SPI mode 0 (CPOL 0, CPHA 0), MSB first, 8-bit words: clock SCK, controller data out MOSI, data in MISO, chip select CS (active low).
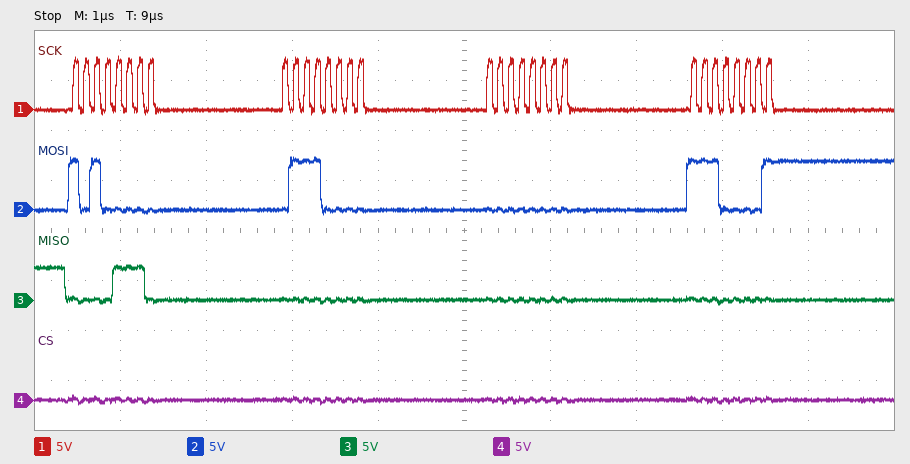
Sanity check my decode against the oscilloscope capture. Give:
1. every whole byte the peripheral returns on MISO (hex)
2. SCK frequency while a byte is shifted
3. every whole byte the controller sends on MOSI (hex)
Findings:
0E 00 00 00
8 MHz
A0 70 00 E1
